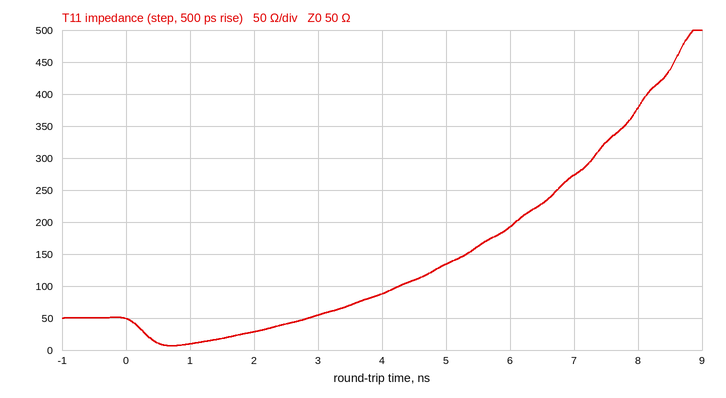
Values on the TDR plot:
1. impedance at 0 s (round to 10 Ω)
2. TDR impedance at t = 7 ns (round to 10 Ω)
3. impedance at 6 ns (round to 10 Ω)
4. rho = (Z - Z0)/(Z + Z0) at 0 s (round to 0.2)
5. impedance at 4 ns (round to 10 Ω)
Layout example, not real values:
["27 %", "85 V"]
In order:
["50 Ω", "270 Ω", "190 Ω", "0.0", "90 Ω"]
